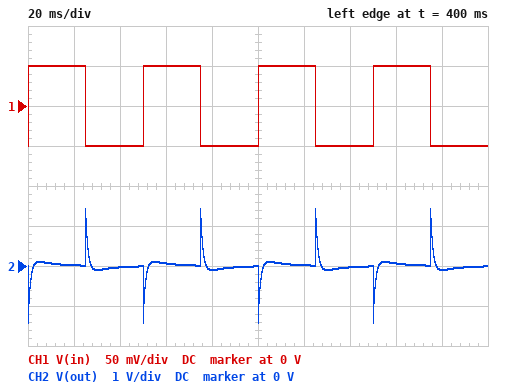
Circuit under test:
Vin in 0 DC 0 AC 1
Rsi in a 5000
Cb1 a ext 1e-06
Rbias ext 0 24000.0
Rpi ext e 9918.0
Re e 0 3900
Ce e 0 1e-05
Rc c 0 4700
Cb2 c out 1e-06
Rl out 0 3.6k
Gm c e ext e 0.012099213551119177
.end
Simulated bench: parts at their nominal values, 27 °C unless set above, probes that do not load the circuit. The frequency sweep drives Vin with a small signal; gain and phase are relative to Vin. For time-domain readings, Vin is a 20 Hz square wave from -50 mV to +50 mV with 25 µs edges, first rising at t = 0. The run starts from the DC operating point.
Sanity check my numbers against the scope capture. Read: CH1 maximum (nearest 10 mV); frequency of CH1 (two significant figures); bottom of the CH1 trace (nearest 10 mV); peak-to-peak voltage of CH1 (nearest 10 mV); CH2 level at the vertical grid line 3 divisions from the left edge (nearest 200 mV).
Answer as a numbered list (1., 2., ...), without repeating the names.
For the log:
1. 50 mV
2. 20 Hz
3. -50 mV
4. 100 mV
5. 0 V
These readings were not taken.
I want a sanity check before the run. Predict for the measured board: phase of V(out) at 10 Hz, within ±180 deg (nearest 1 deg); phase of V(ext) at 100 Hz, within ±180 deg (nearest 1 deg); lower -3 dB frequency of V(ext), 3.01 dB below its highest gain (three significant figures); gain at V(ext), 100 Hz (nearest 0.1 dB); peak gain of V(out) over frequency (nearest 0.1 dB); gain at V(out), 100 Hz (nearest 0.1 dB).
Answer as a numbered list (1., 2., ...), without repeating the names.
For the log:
1. -25 deg
2. -4 deg
3. 5.17 Hz
4. -2.8 dB
5. 23.2 dB
6. 17.9 dB
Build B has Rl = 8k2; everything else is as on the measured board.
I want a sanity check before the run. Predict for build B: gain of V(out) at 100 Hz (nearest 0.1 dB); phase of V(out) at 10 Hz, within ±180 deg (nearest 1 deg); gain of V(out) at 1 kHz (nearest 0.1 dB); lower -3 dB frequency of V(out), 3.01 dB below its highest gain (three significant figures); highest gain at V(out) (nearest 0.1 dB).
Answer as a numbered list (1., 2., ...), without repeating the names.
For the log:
1. 21.3 dB
2. -37 deg
3. 26.4 dB
4. 150 Hz
5. 26.5 dB
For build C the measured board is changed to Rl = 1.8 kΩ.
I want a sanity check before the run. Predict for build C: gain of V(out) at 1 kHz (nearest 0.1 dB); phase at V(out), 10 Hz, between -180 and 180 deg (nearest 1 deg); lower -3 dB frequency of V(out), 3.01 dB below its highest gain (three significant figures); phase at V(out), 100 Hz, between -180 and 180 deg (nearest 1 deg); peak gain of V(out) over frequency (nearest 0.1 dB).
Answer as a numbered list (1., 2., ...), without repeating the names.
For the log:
1. 19.2 dB
2. -20 deg
3. 153 Hz
4. -109 deg
5. 19.3 dB
